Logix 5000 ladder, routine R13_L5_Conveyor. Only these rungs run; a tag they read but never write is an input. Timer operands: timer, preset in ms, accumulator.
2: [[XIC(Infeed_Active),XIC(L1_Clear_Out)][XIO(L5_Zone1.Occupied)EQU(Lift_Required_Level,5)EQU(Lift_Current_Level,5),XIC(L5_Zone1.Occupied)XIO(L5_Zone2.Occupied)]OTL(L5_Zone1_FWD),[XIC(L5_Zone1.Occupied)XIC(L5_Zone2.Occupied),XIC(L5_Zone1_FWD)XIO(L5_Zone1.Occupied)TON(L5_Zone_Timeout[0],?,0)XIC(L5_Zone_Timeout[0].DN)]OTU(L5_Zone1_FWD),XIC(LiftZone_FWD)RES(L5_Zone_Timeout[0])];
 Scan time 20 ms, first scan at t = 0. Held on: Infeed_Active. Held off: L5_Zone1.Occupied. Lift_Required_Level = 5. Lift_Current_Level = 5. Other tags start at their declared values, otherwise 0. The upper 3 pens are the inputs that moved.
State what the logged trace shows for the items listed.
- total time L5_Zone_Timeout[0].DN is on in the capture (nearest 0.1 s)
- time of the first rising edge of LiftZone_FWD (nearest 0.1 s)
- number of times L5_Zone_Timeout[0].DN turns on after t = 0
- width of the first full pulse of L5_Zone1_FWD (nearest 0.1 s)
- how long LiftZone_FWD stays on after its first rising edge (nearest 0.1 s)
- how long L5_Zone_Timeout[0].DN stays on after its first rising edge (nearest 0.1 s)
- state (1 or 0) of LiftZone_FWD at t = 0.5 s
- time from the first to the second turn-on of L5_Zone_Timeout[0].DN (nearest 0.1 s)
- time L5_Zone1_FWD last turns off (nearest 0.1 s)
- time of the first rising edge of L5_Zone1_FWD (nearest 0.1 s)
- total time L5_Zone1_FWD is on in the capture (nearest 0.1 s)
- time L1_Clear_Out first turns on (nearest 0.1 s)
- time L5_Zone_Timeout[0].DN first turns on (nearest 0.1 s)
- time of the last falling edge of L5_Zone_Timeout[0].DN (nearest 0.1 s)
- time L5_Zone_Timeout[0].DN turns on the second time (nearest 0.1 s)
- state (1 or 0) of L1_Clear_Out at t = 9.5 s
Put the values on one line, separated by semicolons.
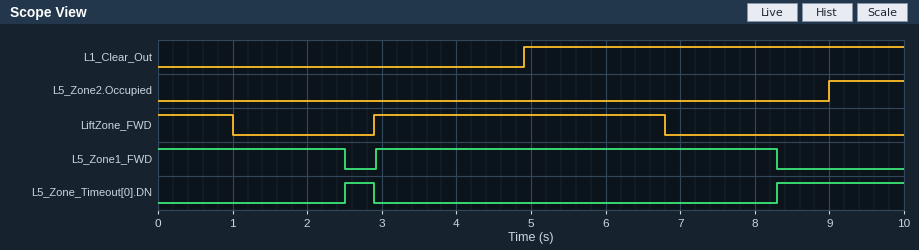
2.1 s; 2.9 s; 2; 5.4 s; 3.9 s; 0.4 s; 1; 5.8 s; 8.3 s; 2.9 s; 7.9 s; 4.9 s; 2.5 s; 2.9 s; 8.3 s; 1
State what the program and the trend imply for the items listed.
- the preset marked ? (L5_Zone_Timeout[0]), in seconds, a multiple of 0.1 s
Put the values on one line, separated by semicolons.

1.5 s
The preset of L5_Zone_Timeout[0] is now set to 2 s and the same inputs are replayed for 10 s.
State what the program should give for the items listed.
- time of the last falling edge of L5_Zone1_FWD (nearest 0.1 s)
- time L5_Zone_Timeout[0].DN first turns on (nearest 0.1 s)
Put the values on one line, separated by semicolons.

8.8 s; 8.8 s
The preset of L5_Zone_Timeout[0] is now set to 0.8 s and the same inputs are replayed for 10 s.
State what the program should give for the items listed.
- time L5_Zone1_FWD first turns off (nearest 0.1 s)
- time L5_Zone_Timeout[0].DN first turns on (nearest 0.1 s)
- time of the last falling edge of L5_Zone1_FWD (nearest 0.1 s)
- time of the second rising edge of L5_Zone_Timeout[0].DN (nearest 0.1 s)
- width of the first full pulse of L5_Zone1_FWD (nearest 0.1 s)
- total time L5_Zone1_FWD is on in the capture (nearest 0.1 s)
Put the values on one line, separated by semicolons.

1.8 s; 1.8 s; 7.6 s; 7.6 s; 4.7 s; 6.5 s
